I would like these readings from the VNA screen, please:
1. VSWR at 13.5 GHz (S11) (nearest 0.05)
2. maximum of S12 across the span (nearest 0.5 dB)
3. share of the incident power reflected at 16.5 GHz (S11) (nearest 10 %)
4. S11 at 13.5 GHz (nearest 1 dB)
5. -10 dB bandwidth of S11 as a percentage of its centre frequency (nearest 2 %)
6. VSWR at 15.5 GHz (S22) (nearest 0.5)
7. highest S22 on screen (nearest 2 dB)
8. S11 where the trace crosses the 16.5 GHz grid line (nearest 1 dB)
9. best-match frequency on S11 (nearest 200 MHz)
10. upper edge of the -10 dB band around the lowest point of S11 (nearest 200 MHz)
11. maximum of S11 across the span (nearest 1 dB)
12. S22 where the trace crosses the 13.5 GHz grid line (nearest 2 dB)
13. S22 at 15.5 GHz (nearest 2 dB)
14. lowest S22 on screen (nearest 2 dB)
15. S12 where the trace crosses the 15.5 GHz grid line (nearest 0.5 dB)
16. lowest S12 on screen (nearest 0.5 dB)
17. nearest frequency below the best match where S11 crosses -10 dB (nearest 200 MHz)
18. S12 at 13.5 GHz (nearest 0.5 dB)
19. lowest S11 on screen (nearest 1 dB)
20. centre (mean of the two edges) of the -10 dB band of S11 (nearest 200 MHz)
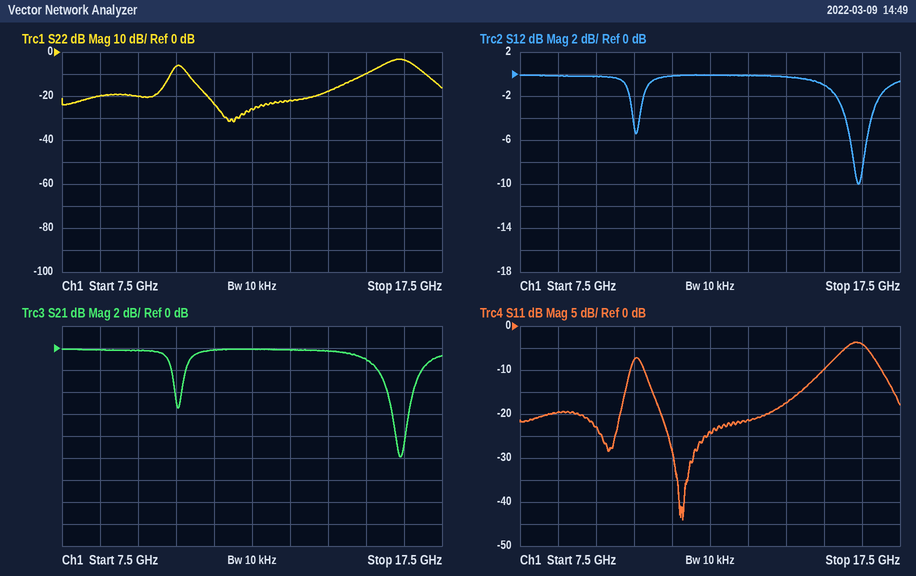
1.20
0.0 dB
40 %
-21 dB
36 %
2.0
-4 dB
-4 dB
11.8 GHz
15.4 GHz
-4 dB
-22 dB
-10 dB
-32 dB
-1.0 dB
-10.0 dB
10.8 GHz
0.0 dB
-44 dB
13.2 GHz
